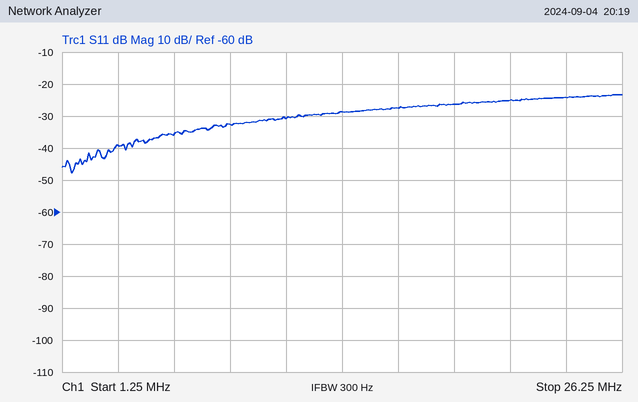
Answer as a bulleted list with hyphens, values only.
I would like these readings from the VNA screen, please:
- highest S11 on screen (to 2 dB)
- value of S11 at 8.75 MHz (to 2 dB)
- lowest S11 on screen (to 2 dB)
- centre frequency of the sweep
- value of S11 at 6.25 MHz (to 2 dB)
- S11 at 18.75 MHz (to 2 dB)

- -24 dB
- -32 dB
- -48 dB
- 13.75 MHz
- -36 dB
- -26 dB
